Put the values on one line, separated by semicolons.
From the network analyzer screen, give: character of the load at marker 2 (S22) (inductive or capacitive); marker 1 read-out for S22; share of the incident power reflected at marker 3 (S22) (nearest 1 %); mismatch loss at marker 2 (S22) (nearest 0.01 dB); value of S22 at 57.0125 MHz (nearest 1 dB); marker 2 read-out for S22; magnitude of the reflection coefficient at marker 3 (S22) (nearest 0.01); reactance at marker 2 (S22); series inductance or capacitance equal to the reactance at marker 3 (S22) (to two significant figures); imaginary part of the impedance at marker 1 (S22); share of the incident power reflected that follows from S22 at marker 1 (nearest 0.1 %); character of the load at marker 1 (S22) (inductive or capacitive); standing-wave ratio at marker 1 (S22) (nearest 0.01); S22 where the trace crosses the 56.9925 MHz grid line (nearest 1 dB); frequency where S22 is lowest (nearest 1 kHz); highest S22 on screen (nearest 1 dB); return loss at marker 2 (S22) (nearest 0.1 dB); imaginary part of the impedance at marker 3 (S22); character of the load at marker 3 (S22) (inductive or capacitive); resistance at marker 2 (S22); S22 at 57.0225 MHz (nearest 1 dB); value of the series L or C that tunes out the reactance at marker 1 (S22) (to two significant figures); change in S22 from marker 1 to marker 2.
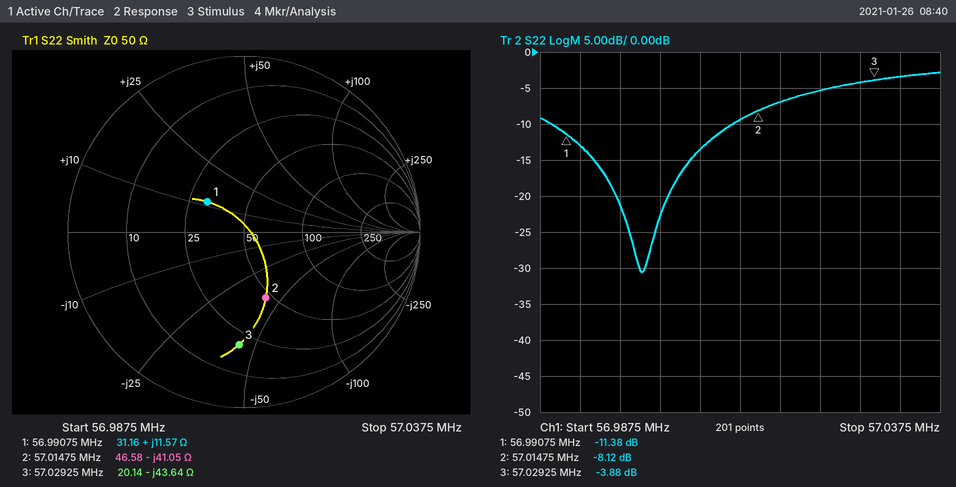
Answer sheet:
capacitive; -11.38 dB; 41 %; 0.73 dB; -9 dB; -8.12 dB; 0.64; -41.05 Ω; 64 pF; +11.57 Ω; 7.3 %; inductive; 1.74; -13 dB; 57.000 MHz; -3 dB; 8.1 dB; -43.64 Ω; capacitive; 46.58 Ω; -5 dB; 240 pF; 3.26 dB
